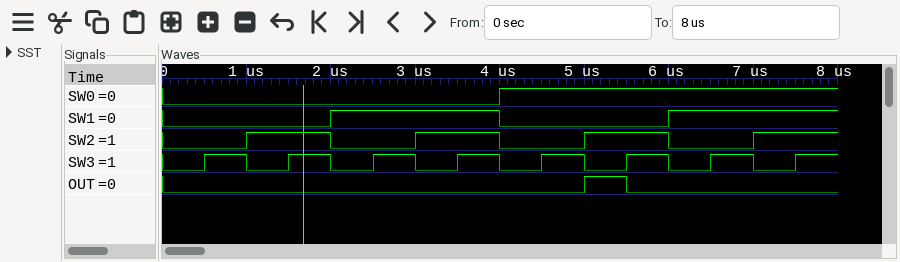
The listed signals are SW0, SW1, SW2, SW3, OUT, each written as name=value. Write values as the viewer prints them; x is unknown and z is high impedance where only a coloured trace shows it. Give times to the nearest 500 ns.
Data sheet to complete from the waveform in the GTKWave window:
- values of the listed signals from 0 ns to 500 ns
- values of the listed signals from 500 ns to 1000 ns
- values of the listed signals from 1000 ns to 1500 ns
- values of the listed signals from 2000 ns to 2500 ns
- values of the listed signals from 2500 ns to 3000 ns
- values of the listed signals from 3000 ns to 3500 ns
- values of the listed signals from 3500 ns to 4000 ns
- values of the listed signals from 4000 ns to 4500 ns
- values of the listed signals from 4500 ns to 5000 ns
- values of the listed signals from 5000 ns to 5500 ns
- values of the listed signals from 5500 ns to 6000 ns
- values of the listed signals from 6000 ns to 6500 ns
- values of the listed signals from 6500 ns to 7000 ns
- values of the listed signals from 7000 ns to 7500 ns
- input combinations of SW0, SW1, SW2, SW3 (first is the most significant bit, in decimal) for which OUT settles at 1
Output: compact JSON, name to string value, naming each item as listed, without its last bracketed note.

{"values of the listed signals from 0 ns to 500 ns": "SW0=0, SW1=0, SW2=0, SW3=0, OUT=0", "values of the listed signals from 500 ns to 1000 ns": "SW0=0, SW1=0, SW2=0, SW3=1, OUT=0", "values of the listed signals from 1000 ns to 1500 ns": "SW0=0, SW1=0, SW2=1, SW3=0, OUT=0", "values of the listed signals from 2000 ns to 2500 ns": "SW0=0, SW1=1, SW2=0, SW3=0, OUT=0", "values of the listed signals from 2500 ns to 3000 ns": "SW0=0, SW1=1, SW2=0, SW3=1, OUT=0", "values of the listed signals from 3000 ns to 3500 ns": "SW0=0, SW1=1, SW2=1, SW3=0, OUT=0", "values of the listed signals from 3500 ns to 4000 ns": "SW0=0, SW1=1, SW2=1, SW3=1, OUT=0", "values of the listed signals from 4000 ns to 4500 ns": "SW0=1, SW1=0, SW2=0, SW3=0, OUT=0", "values of the listed signals from 4500 ns to 5000 ns": "SW0=1, SW1=0, SW2=0, SW3=1, OUT=0", "values of the listed signals from 5000 ns to 5500 ns": "SW0=1, SW1=0, SW2=1, SW3=0, OUT=1", "values of the listed signals from 5500 ns to 6000 ns": "SW0=1, SW1=0, SW2=1, SW3=1, OUT=0", "values of the listed signals from 6000 ns to 6500 ns": "SW0=1, SW1=1, SW2=0, SW3=0, OUT=0", "values of the listed signals from 6500 ns to 7000 ns": "SW0=1, SW1=1, SW2=0, SW3=1, OUT=0", "values of the listed signals from 7000 ns to 7500 ns": "SW0=1, SW1=1, SW2=1, SW3=0, OUT=0", "input combinations of SW0, SW1, SW2, SW3 (first is the most significant bit, in decimal) for which OUT settles at 1": "10"}
